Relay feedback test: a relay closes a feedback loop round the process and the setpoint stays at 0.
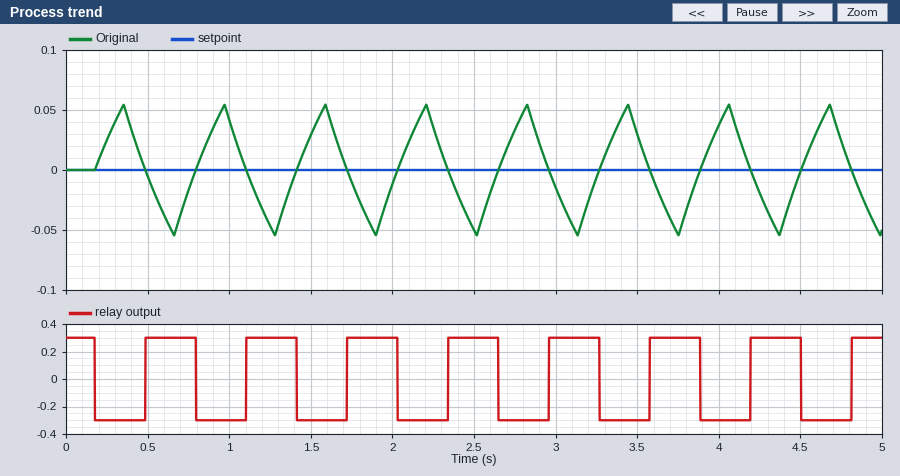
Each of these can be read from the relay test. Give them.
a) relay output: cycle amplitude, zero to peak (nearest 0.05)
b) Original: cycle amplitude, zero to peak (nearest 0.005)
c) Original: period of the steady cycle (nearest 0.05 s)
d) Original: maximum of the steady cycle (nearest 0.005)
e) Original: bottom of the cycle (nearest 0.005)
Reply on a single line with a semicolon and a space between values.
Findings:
0.30; 0.055; 0.60 s; 0.055; -0.055
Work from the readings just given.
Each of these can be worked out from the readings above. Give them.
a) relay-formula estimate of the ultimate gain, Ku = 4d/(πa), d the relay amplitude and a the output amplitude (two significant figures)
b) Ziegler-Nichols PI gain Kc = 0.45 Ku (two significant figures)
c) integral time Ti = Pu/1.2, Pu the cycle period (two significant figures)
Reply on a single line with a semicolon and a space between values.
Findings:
6.9; 3.1; 0.50 s
